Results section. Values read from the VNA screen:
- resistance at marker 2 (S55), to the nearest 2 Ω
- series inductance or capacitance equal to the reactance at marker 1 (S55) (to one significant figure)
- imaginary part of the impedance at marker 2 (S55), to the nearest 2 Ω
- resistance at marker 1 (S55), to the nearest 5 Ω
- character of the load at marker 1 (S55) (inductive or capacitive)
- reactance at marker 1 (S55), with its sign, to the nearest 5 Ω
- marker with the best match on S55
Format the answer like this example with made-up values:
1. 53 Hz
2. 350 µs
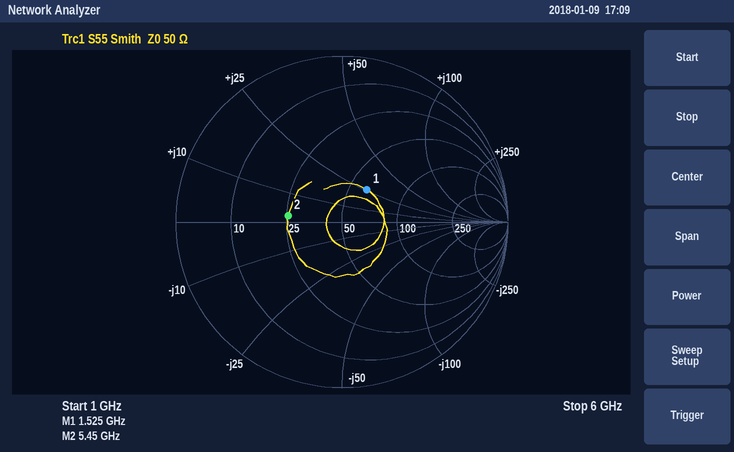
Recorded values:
1. 26 Ω
2. 3 nH
3. +2 Ω
4. 60 Ω
5. inductive
6. +25 Ω
7. marker 1
